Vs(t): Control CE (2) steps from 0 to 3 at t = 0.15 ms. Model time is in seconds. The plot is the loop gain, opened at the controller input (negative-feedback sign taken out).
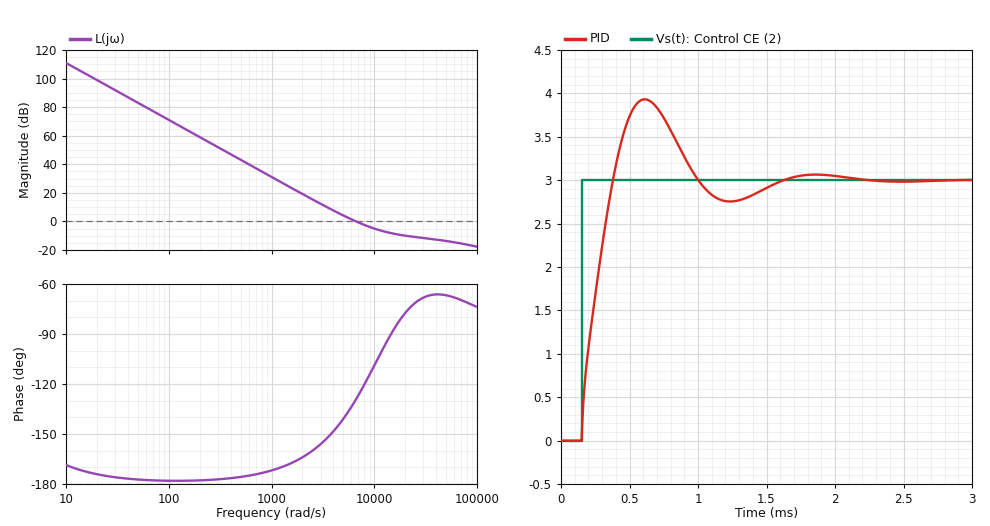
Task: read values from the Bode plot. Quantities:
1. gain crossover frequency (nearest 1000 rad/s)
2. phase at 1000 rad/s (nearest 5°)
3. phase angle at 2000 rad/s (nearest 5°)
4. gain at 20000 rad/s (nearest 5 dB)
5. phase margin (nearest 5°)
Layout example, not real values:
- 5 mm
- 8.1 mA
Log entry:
- 7000 rad/s
- -170°
- -165°
- -10 dB
- 50°
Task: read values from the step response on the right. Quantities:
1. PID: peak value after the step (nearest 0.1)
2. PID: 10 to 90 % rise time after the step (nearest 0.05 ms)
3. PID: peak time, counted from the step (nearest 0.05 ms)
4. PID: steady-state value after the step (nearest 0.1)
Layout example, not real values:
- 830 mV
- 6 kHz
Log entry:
- 3.9
- 0.20 ms
- 0.45 ms
- 3.0
